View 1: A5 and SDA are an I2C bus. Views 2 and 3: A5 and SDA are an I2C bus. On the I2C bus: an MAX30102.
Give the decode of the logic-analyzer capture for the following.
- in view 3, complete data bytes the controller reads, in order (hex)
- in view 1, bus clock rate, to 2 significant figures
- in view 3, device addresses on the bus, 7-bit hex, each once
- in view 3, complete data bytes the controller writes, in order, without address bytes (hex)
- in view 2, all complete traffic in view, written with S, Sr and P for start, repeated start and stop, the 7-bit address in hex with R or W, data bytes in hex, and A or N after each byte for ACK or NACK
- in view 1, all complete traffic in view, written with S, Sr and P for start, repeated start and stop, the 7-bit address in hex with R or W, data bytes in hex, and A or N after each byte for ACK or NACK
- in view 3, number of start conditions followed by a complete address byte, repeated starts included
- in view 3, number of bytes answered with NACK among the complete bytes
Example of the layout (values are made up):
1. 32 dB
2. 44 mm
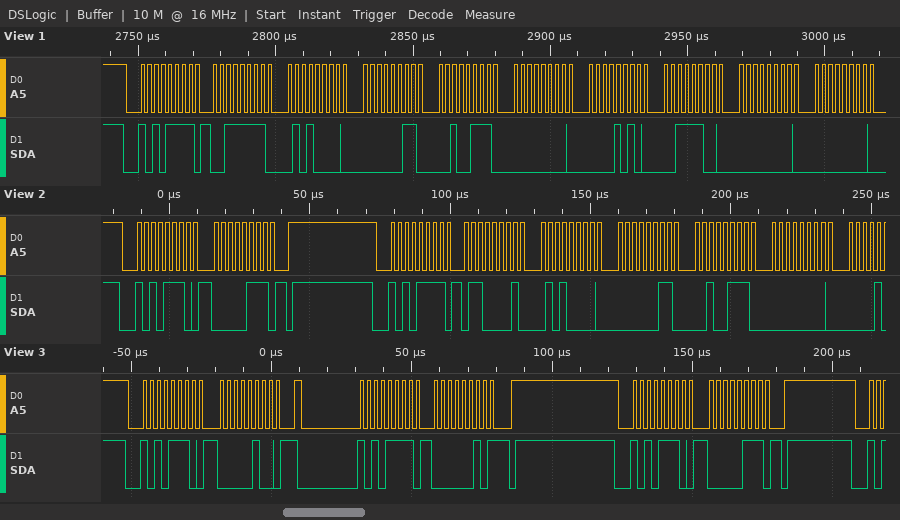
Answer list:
1. 02
2. 400 kHz
3. 0x57
4. 04 07
5. S 57W A 07 A P S 57R A 61 A 50 A 03 A 27 A 00 A
6. S 57R A 3F A 50 A 03 A 27 A 00 A 0A A 3C A 00 A 00 A
7. 3
8. 1
